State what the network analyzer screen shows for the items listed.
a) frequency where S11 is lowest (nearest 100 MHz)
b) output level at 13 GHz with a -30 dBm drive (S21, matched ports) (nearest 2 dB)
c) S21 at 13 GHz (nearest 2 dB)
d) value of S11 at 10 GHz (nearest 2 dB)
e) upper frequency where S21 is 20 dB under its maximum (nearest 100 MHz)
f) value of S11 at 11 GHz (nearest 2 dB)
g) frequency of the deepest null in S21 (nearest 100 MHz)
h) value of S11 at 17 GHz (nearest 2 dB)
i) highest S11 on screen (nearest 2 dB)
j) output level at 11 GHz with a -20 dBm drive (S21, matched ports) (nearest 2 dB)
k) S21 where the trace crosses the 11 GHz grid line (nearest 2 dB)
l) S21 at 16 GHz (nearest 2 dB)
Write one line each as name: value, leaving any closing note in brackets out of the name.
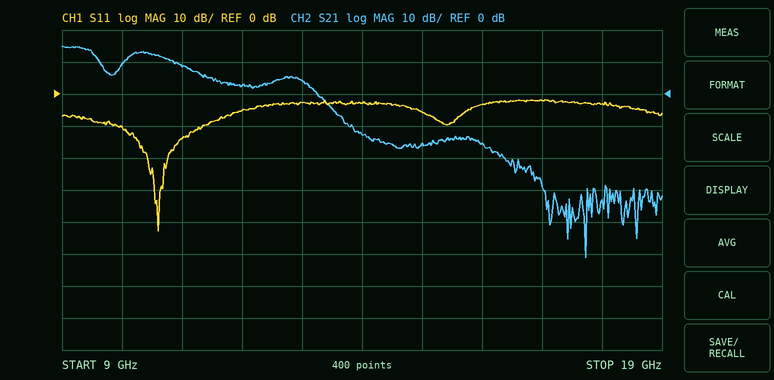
frequency where S11 is lowest: 10.6 GHz
output level at 13 GHz with a -30 dBm drive (S21, matched ports): -26 dBm
S21 at 13 GHz: 4 dB
value of S11 at 10 GHz: -10 dB
upper frequency where S21 is 20 dB under its maximum: 13.5 GHz
value of S11 at 11 GHz: -14 dB
frequency of the deepest null in S21: 17.7 GHz
value of S11 at 17 GHz: -2 dB
highest S11 on screen: -2 dB
output level at 11 GHz with a -20 dBm drive (S21, matched ports): -12 dBm
S21 where the trace crosses the 11 GHz grid line: 8 dB
S21 at 16 GHz: -16 dB
